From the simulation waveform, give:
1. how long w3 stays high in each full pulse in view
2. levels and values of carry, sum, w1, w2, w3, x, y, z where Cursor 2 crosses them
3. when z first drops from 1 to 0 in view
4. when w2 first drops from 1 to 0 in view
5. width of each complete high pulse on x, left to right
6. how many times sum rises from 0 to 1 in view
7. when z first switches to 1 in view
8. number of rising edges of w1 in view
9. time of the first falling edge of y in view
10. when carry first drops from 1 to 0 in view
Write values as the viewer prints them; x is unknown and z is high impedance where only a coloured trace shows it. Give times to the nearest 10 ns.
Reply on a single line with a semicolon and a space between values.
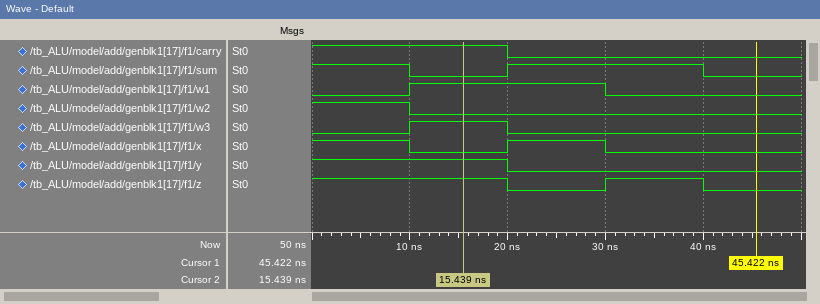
10 ns; carry=1, sum=0, w1=1, w2=0, w3=1, x=0, y=1, z=1; 20 ns; 10 ns; 10 ns; 1; 30 ns; 1; 20 ns; 20 ns
